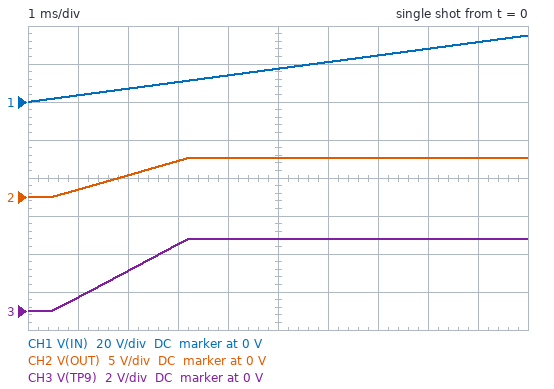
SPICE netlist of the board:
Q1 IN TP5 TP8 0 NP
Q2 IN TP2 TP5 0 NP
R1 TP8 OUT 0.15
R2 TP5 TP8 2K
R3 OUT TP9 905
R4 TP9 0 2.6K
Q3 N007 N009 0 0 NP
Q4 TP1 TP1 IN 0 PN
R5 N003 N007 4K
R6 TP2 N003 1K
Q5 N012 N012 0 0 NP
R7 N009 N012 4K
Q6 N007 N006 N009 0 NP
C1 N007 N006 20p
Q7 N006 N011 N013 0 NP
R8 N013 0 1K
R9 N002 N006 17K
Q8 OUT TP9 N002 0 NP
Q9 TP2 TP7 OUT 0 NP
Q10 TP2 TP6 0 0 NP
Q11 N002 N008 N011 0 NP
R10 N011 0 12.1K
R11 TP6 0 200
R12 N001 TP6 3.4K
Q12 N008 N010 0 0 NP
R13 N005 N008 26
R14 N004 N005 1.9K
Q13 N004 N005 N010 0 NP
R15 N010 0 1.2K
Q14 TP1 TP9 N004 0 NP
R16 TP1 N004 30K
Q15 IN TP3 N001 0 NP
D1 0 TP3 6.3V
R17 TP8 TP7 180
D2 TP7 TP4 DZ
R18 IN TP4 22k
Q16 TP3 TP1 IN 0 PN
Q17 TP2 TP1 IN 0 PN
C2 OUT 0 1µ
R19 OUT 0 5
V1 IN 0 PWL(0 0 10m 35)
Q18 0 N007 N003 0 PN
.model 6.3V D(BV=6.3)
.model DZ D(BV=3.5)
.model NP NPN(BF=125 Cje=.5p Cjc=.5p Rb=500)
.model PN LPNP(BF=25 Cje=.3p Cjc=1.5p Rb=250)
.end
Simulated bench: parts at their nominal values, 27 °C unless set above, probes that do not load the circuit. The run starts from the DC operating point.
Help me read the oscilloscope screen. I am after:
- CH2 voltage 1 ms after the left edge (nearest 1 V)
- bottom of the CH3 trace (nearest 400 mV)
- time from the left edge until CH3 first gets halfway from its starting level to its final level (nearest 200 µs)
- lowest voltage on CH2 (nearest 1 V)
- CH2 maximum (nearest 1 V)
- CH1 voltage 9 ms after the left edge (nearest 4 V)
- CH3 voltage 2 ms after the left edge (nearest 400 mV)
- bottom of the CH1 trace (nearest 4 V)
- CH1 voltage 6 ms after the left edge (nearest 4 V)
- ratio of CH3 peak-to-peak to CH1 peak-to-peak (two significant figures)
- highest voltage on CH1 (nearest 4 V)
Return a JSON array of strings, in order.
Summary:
["1 V", "0 V", "1.8 ms", "0 V", "5 V", "32 V", "2.0 V", "0 V", "20 V", "0.11", "36 V"]
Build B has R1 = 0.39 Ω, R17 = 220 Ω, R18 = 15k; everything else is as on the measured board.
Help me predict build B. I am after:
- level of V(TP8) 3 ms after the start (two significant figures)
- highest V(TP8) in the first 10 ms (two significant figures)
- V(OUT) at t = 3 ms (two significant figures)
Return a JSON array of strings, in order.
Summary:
["5.0 V", "5.5 V", "4.6 V"]
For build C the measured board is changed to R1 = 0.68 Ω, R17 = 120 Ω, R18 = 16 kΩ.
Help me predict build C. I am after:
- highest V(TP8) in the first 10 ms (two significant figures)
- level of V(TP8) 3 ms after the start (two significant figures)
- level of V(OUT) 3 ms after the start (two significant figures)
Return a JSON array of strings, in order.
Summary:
["5.8 V", "5.1 V", "4.5 V"]
